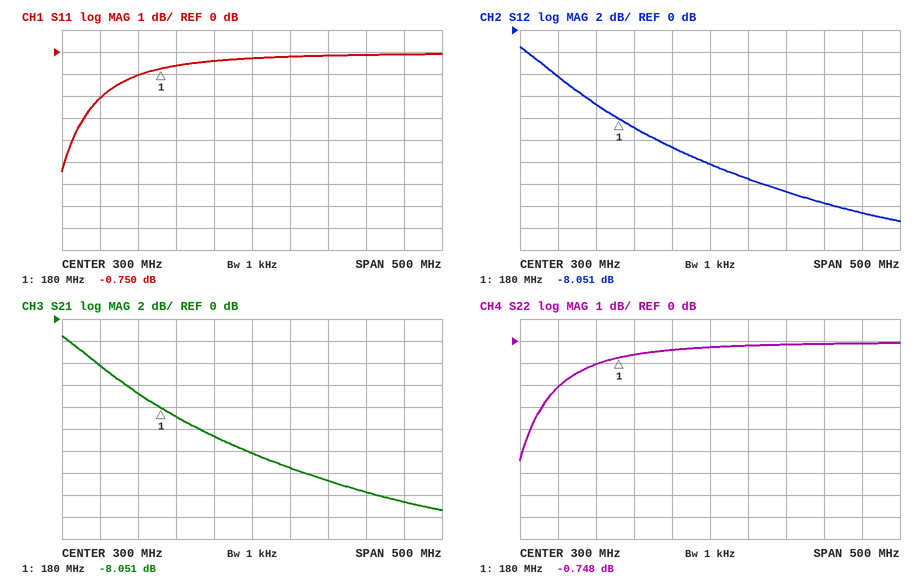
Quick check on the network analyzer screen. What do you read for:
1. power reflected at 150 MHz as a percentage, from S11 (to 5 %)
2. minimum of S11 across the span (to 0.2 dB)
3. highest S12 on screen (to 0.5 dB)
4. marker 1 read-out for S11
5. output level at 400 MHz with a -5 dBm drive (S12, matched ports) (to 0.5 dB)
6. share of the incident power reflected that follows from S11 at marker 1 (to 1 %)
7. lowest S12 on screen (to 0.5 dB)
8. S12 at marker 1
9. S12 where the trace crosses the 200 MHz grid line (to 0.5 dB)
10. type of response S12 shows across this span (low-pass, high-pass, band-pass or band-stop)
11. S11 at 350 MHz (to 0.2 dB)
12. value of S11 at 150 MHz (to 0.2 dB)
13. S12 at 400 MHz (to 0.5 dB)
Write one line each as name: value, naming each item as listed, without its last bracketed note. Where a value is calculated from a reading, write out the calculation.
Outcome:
power reflected at 150 MHz as a percentage, from S11: 10^(-1/10) ≈ 79.4 %, so 80 % to the nearest 5 %
minimum of S11 across the span: -5.4 dB
highest S12 on screen: -1.5 dB
marker 1 read-out for S11: -0.750 dB
output level at 400 MHz with a -5 dBm drive (S12, matched ports): -5 dBm + (-14.5 dB) = -19.5 dBm
share of the incident power reflected that follows from S11 at marker 1: 10^(-0.75/10) ≈ 84 %
lowest S12 on screen: -17.5 dB
S12 at marker 1: -8.051 dB
S12 where the trace crosses the 200 MHz grid line: -9.0 dB
type of response S12 shows across this span: low-pass
S11 at 350 MHz: -0.2 dB
value of S11 at 150 MHz: -1.0 dB
S12 at 400 MHz: -14.5 dB
